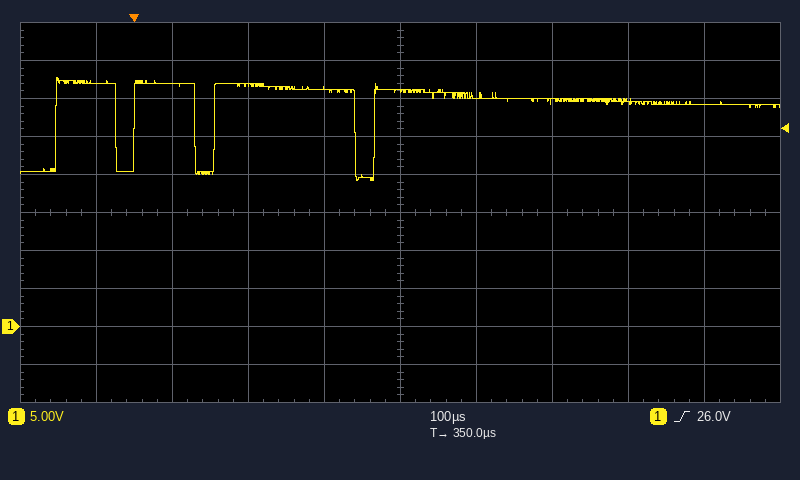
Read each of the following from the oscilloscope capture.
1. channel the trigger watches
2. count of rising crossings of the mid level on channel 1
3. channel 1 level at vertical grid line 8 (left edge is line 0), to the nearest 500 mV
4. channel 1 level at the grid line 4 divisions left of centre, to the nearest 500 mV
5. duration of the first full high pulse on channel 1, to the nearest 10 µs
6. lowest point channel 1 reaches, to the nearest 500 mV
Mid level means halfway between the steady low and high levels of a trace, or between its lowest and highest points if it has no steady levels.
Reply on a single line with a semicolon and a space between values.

channel 1; 4; 29.5 V; 32.0 V; 80 µs; 19.0 V
